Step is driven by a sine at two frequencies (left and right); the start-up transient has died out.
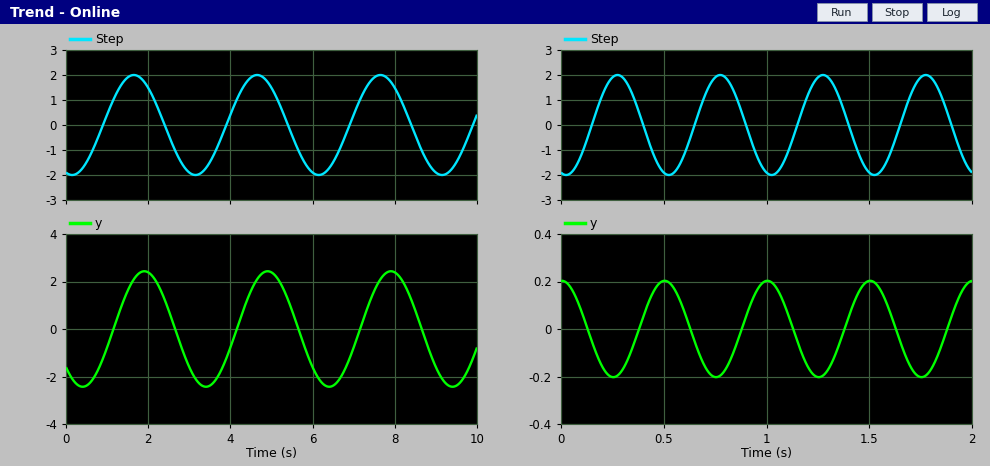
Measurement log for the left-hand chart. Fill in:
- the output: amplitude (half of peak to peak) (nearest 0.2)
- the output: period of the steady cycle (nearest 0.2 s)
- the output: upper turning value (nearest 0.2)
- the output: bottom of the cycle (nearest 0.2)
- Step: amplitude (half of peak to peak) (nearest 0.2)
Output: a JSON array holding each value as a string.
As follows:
["2.4", "3.0 s", "2.4", "-2.4", "2.0"]
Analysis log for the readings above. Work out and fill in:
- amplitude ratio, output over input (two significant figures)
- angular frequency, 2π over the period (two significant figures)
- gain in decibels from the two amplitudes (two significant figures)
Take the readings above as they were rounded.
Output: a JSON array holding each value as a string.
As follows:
["1.2", "2.1 rad/s", "1.6 dB"]
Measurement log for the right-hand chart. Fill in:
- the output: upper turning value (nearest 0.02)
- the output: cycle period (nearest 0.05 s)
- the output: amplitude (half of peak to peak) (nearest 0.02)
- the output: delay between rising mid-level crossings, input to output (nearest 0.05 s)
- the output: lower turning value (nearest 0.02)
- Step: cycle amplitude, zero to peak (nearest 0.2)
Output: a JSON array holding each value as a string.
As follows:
["0.20", "0.50 s", "0.20", "0.25 s", "-0.20", "2.0"]
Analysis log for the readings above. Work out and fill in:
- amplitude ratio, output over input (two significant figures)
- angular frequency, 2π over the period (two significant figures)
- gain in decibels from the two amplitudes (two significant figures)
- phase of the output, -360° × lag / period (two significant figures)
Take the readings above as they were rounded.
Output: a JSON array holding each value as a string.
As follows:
["0.10", "13 rad/s", "-20 dB", "-180°"]
